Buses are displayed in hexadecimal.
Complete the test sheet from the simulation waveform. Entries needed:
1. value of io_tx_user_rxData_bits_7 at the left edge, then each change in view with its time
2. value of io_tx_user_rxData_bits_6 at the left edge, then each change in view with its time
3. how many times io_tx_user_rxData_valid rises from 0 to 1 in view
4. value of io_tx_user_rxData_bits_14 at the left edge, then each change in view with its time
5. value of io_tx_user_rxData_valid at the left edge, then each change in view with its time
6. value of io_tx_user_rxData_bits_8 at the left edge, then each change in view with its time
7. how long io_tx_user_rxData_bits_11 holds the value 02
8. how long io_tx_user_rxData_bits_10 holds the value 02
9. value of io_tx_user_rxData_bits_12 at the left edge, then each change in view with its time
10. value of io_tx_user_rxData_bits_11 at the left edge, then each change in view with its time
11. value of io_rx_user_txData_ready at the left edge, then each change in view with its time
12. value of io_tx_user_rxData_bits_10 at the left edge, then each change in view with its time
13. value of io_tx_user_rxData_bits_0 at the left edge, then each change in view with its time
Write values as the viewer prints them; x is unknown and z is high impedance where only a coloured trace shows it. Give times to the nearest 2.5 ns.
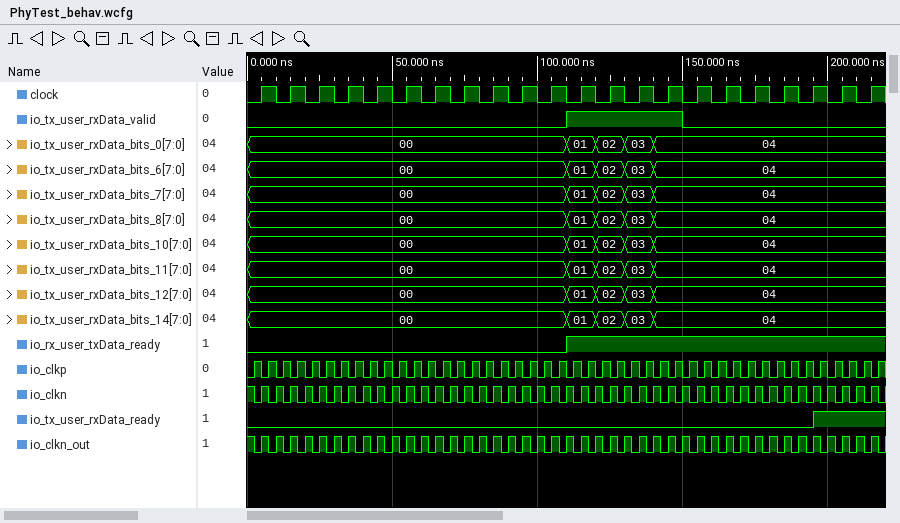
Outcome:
00, 01 at 110 ns, 02 at 120 ns, 03 at 130 ns, 04 at 140 ns
00, 01 at 110 ns, 02 at 120 ns, 03 at 130 ns, 04 at 140 ns
1
00, 01 at 110 ns, 02 at 120 ns, 03 at 130 ns, 04 at 140 ns
0, 1 at 110 ns, 0 at 150 ns
00, 01 at 110 ns, 02 at 120 ns, 03 at 130 ns, 04 at 140 ns
10 ns
10 ns
00, 01 at 110 ns, 02 at 120 ns, 03 at 130 ns, 04 at 140 ns
00, 01 at 110 ns, 02 at 120 ns, 03 at 130 ns, 04 at 140 ns
0, 1 at 110 ns
00, 01 at 110 ns, 02 at 120 ns, 03 at 130 ns, 04 at 140 ns
00, 01 at 110 ns, 02 at 120 ns, 03 at 130 ns, 04 at 140 ns
